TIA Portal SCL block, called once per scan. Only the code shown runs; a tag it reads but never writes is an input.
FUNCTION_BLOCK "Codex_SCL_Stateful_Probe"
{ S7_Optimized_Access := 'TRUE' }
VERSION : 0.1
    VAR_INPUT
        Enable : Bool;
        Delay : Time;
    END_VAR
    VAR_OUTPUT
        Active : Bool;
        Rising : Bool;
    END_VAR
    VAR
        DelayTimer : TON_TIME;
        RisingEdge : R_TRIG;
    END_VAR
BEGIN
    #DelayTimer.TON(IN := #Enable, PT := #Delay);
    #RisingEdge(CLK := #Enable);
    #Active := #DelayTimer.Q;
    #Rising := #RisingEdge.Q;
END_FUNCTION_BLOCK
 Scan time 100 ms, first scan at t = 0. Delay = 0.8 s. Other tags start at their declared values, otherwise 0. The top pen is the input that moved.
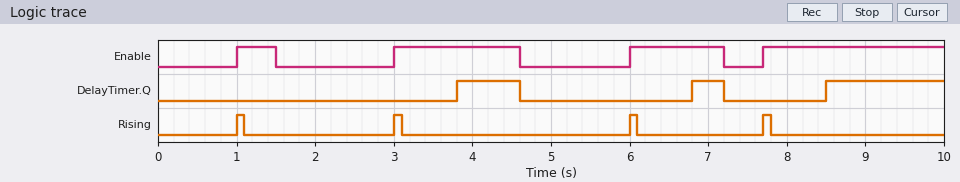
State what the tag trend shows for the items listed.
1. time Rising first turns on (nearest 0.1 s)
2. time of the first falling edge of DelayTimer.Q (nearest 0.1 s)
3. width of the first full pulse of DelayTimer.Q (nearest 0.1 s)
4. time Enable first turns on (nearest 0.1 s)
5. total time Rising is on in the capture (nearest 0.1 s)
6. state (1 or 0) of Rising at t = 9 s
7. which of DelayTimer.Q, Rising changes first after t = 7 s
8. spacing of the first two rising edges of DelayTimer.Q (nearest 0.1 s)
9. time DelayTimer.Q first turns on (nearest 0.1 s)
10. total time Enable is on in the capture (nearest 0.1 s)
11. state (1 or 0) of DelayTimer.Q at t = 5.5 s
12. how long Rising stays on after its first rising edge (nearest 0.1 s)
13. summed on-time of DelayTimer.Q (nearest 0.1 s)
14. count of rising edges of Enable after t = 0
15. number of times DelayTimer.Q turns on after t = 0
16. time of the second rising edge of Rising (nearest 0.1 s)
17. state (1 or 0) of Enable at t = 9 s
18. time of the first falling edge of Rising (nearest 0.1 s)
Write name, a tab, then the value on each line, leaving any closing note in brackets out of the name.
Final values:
time Rising first turns on	1.0 s
time of the first falling edge of DelayTimer.Q	4.6 s
width of the first full pulse of DelayTimer.Q	0.8 s
time Enable first turns on	1.0 s
total time Rising is on in the capture	0.4 s
state (1 or 0) of Rising at t = 9 s	0
which of DelayTimer.Q, Rising changes first after t = 7 s	DelayTimer.Q
spacing of the first two rising edges of DelayTimer.Q	3.0 s
time DelayTimer.Q first turns on	3.8 s
total time Enable is on in the capture	5.6 s
state (1 or 0) of DelayTimer.Q at t = 5.5 s	0
how long Rising stays on after its first rising edge	0.1 s
summed on-time of DelayTimer.Q	2.7 s
count of rising edges of Enable after t = 0	4
number of times DelayTimer.Q turns on after t = 0	3
time of the second rising edge of Rising	3.0 s
state (1 or 0) of Enable at t = 9 s	1
time of the first falling edge of Rising	1.1 s
